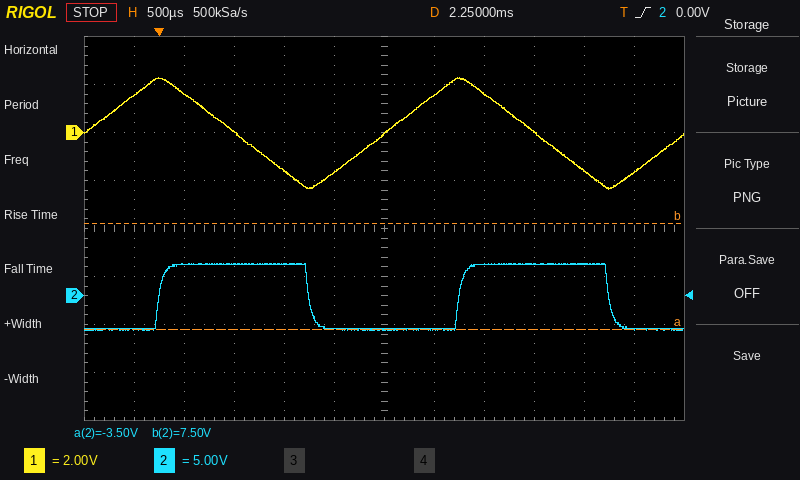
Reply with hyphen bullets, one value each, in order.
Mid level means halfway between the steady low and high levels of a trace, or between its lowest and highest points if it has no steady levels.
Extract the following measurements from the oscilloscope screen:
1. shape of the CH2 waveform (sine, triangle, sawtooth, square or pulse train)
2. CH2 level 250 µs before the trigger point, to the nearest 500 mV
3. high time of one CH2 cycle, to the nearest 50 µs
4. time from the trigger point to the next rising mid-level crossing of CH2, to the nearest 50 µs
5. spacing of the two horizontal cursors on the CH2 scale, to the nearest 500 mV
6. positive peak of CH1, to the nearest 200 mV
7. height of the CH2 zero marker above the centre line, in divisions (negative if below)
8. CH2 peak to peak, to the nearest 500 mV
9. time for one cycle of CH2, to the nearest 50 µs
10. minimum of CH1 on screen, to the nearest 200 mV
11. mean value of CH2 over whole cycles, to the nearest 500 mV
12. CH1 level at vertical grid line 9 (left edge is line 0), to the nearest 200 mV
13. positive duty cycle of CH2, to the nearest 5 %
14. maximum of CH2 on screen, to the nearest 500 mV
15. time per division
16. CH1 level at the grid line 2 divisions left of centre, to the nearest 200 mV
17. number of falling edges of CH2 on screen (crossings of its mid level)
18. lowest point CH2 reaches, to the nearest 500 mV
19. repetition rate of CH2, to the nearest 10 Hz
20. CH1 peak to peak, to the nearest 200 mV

- square
- -3.5 V
- 1.50 ms
- 3.00 ms
- 11.0 V
- 2.2 V
- -1.4 div
- 7.0 V
- 3.00 ms
- -2.4 V
- 0.0 V
- 0.0 V
- 50 %
- 3.5 V
- 500 µs
- -1.6 V
- 2
- -3.5 V
- 330 Hz
- 4.6 V
